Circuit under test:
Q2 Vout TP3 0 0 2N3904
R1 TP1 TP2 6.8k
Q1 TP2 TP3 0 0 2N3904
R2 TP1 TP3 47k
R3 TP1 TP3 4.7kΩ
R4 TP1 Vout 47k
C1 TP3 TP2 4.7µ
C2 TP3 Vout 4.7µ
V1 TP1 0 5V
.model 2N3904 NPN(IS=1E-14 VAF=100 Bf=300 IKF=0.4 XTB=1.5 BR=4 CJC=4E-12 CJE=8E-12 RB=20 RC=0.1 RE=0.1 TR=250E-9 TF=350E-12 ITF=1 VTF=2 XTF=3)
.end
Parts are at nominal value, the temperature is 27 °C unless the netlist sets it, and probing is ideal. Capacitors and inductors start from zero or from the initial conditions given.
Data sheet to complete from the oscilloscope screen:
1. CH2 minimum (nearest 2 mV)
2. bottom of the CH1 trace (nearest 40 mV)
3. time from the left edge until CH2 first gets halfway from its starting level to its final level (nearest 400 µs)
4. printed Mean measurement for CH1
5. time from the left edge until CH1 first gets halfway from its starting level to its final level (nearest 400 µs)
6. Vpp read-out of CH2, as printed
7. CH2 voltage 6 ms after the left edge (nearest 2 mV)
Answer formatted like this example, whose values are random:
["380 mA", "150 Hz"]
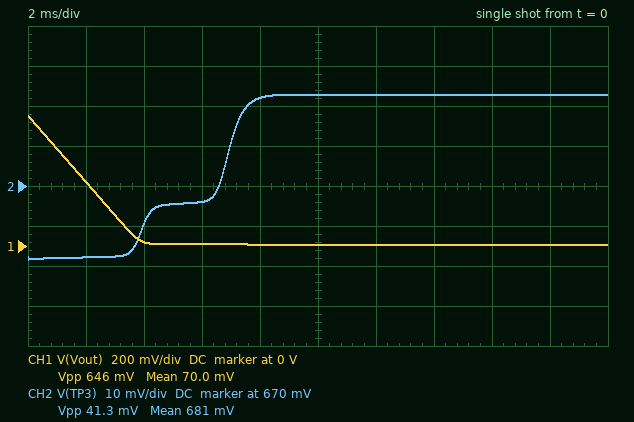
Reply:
["652 mV", "0 V", "6.8 ms", "70.0 mV", "2.0 ms", "41.3 mV", "666 mV"]
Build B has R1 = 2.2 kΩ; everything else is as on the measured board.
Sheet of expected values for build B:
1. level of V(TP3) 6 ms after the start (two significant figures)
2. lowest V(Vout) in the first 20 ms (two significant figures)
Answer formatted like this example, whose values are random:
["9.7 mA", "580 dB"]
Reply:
["680 mV", "6.8 mV"]
